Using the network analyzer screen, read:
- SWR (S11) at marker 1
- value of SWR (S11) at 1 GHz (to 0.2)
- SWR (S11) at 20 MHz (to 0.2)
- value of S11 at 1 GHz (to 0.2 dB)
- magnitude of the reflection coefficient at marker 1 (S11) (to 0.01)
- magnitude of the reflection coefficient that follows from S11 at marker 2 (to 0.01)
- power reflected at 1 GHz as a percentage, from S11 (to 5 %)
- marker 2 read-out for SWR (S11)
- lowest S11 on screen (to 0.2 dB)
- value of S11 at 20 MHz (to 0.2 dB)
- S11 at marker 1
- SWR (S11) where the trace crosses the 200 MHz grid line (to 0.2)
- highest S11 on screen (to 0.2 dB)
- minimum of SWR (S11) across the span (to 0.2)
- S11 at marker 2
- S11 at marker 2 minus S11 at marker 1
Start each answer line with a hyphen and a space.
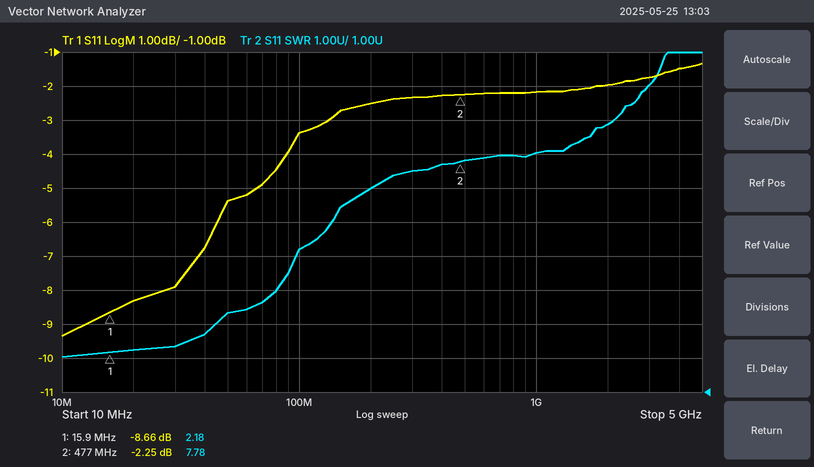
- 2.18
- 8.0
- 2.2
- -2.2 dB
- 0.37
- 0.77
- 60 %
- 7.78
- -9.4 dB
- -8.4 dB
- -8.66 dB
- 7.0
- -1.4 dB
- 2.0
- -2.25 dB
- 6.41 dB
